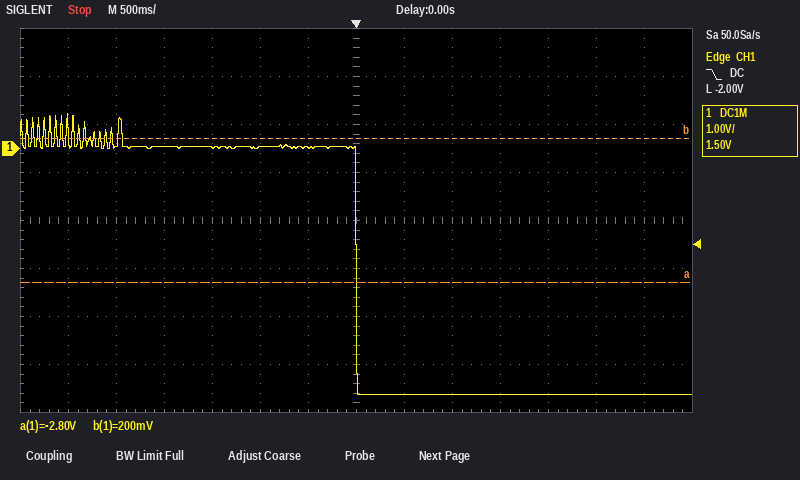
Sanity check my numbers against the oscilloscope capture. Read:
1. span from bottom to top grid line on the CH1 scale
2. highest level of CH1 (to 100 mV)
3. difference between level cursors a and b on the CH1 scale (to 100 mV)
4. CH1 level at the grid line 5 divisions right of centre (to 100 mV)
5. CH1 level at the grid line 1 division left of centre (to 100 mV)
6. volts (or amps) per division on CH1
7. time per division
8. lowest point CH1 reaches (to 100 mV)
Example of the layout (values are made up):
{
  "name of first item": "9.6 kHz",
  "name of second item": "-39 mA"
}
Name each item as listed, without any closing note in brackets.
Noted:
{
  "span from bottom to top grid line on the CH1 scale": "8 V",
  "highest level of CH1": "700 mV",
  "difference between level cursors a and b on the CH1 scale": "3.0 V",
  "CH1 level at the grid line 5 divisions right of centre": "-5.1 V",
  "CH1 level at the grid line 1 division left of centre": "0.0 V",
  "volts (or amps) per division on CH1": "1 V",
  "time per division": "500 ms",
  "lowest point CH1 reaches": "-5.1 V"
}
